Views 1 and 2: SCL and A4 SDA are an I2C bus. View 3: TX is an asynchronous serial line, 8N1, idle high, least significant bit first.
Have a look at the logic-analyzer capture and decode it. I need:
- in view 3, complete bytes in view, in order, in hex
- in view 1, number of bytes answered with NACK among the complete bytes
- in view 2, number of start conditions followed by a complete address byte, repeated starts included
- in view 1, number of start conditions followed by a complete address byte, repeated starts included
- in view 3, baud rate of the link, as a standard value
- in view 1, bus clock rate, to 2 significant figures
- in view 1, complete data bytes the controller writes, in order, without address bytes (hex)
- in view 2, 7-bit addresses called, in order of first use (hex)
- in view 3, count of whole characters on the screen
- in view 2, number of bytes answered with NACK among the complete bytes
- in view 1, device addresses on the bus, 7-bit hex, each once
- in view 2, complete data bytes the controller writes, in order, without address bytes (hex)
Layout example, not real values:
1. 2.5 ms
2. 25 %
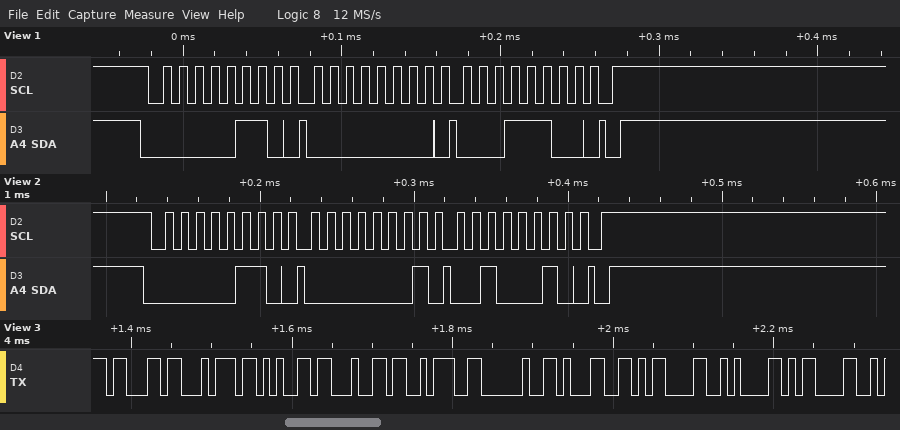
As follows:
1. 63 74 65 64 3A 20 31 0D 0A 0D
2. 0
3. 1
4. 1
5. 115200 baud
6. 100 kHz
7. 00 1C
8. 0x03
9. 10
10. 0
11. 0x03
12. 01 22
